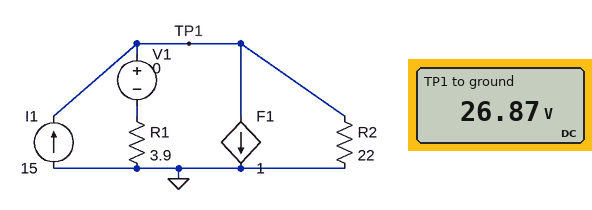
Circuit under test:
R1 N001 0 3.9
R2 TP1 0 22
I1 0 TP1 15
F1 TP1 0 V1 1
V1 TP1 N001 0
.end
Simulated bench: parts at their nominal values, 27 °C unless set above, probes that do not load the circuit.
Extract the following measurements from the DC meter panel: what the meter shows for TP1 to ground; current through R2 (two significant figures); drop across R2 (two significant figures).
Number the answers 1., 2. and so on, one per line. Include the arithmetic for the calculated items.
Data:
1. 26.87 V
2. (26.87 V) / 22 Ω = 1.2 A
3. 26.87 V = 27 V
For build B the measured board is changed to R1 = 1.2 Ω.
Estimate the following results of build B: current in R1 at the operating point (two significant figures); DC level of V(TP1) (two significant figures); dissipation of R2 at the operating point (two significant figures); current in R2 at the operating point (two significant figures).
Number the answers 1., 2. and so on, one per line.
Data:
1. 7.3 A
2. 8.8 V
3. 3.5 W
4. 400 mA
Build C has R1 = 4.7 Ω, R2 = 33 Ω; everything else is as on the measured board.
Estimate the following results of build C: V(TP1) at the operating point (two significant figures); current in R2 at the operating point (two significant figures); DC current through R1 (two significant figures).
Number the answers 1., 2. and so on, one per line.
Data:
1. 33 V
2. 1.0 A
3. 7.0 A
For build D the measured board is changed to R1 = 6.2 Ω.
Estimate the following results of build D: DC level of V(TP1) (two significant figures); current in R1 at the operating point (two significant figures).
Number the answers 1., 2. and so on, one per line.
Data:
1. 41 V
2. 6.6 A
